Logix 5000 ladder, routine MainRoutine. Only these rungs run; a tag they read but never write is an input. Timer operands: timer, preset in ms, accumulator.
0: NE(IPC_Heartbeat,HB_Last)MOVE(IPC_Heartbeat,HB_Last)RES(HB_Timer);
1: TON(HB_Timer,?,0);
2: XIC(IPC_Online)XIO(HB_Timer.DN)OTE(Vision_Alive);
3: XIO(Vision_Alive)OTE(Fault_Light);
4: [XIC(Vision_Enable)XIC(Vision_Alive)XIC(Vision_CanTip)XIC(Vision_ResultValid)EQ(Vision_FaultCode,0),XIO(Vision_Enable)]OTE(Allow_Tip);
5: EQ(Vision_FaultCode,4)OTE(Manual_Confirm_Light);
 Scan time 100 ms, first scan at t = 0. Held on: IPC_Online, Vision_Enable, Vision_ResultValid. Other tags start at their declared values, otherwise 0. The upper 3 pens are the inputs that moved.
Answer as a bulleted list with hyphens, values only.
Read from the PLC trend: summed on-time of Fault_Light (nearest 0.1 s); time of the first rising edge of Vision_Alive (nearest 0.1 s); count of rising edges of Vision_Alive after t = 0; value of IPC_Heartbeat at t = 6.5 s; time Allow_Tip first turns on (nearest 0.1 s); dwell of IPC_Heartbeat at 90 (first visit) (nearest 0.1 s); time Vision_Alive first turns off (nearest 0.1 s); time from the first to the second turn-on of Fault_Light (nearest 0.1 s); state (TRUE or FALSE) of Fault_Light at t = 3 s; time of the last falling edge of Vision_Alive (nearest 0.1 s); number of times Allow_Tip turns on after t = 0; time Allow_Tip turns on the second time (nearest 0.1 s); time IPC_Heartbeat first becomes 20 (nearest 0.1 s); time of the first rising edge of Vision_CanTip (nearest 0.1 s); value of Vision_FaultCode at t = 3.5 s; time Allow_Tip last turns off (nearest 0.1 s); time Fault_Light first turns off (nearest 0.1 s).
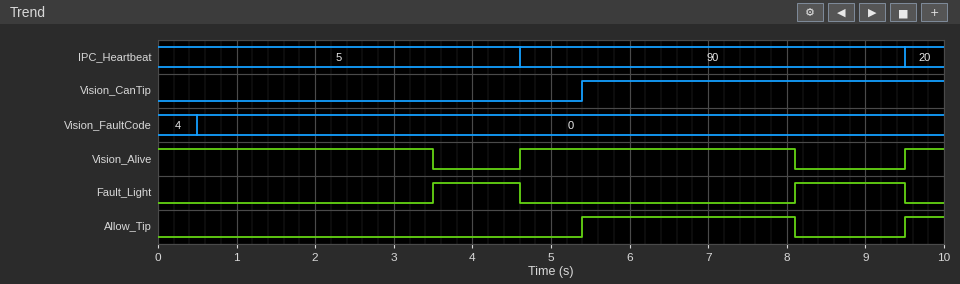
- 2.5 s
- 4.6 s
- 2
- 90
- 5.4 s
- 4.9 s
- 3.5 s
- 4.6 s
- FALSE
- 8.1 s
- 2
- 9.5 s
- 9.5 s
- 5.4 s
- 0
- 8.1 s
- 4.6 s
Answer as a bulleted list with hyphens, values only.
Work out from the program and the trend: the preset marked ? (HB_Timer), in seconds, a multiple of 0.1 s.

- 3.5 s
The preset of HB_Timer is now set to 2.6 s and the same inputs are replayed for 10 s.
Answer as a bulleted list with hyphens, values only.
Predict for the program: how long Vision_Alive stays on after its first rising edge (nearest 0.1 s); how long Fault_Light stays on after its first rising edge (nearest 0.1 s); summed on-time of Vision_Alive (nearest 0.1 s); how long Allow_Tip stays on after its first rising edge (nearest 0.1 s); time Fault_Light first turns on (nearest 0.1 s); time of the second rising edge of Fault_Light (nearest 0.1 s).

- 2.6 s
- 2.0 s
- 5.7 s
- 1.8 s
- 2.6 s
- 7.2 s
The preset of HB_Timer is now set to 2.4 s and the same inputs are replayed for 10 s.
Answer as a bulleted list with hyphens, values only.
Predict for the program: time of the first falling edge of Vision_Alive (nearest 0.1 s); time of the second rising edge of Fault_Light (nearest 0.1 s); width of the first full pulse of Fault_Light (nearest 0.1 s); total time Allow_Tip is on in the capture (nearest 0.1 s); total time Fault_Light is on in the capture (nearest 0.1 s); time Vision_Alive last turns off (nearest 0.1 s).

- 2.4 s
- 7.0 s
- 2.2 s
- 2.1 s
- 4.7 s
- 7.0 s
